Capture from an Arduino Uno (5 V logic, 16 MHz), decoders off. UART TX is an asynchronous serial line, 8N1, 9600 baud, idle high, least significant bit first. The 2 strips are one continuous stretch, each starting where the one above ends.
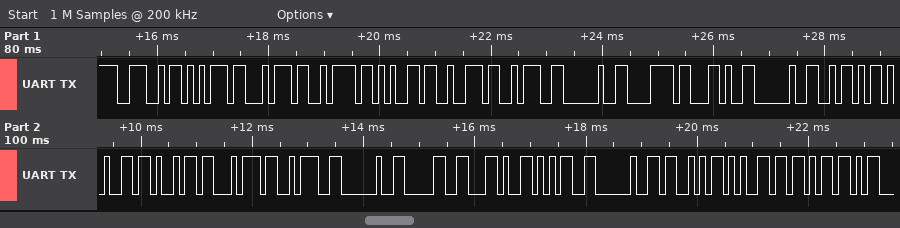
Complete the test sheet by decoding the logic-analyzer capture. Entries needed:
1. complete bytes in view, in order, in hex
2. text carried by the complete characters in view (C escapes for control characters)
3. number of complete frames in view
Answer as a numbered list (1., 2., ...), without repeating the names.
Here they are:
1. 4E 75 74 7A 65 72 3A 20 78 2C 20 5A 65 69 74 3A 20 30 2C 35 20 53 65 6B
2. "Nutzer: x, Zeit: 0,5 Sek"
3. 24
